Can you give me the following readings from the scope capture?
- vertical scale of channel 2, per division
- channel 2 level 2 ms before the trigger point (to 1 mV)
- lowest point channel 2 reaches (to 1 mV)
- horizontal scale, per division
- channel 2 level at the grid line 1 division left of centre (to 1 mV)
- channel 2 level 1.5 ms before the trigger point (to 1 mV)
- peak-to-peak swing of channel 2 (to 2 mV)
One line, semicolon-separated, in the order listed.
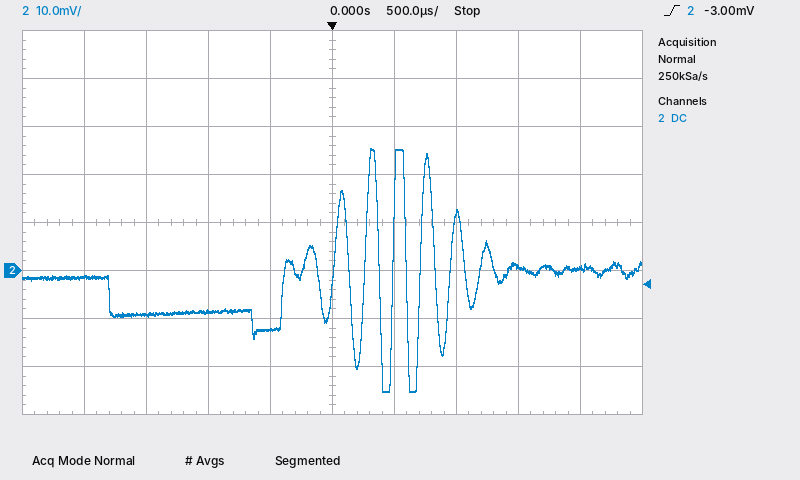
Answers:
10 mV; -1 mV; -25 mV; 500 µs; -12 mV; -9 mV; 50 mV
